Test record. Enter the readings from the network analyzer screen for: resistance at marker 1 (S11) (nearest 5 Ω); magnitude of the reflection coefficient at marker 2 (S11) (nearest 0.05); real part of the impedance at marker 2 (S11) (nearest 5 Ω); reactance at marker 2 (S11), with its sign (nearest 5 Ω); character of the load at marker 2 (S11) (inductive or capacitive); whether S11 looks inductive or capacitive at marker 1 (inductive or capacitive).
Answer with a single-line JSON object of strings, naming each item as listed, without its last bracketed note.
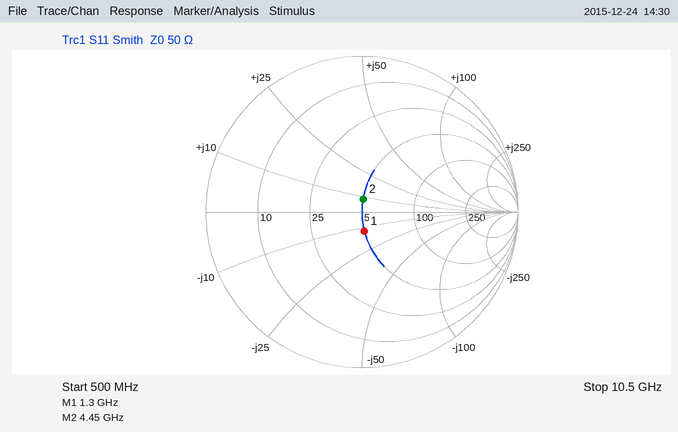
{"resistance at marker 1 (S11)": "50 Ω", "magnitude of the reflection coefficient at marker 2 (S11)": "0.10", "real part of the impedance at marker 2 (S11)": "50 Ω", "reactance at marker 2 (S11), with its sign": "+10 Ω", "character of the load at marker 2 (S11)": "inductive", "whether S11 looks inductive or capacitive at marker 1": "capacitive"}
